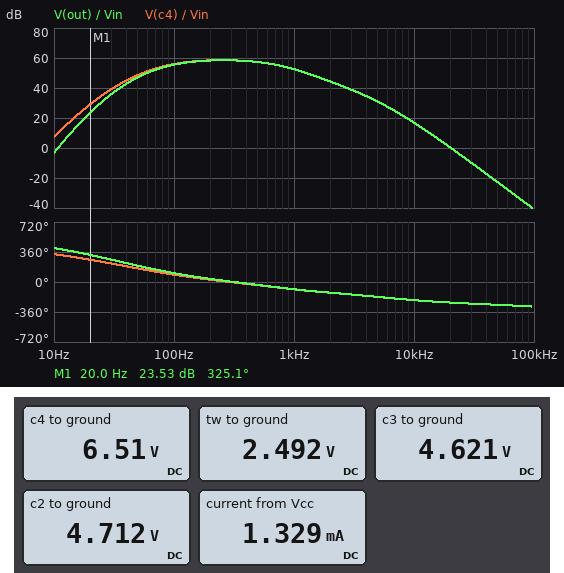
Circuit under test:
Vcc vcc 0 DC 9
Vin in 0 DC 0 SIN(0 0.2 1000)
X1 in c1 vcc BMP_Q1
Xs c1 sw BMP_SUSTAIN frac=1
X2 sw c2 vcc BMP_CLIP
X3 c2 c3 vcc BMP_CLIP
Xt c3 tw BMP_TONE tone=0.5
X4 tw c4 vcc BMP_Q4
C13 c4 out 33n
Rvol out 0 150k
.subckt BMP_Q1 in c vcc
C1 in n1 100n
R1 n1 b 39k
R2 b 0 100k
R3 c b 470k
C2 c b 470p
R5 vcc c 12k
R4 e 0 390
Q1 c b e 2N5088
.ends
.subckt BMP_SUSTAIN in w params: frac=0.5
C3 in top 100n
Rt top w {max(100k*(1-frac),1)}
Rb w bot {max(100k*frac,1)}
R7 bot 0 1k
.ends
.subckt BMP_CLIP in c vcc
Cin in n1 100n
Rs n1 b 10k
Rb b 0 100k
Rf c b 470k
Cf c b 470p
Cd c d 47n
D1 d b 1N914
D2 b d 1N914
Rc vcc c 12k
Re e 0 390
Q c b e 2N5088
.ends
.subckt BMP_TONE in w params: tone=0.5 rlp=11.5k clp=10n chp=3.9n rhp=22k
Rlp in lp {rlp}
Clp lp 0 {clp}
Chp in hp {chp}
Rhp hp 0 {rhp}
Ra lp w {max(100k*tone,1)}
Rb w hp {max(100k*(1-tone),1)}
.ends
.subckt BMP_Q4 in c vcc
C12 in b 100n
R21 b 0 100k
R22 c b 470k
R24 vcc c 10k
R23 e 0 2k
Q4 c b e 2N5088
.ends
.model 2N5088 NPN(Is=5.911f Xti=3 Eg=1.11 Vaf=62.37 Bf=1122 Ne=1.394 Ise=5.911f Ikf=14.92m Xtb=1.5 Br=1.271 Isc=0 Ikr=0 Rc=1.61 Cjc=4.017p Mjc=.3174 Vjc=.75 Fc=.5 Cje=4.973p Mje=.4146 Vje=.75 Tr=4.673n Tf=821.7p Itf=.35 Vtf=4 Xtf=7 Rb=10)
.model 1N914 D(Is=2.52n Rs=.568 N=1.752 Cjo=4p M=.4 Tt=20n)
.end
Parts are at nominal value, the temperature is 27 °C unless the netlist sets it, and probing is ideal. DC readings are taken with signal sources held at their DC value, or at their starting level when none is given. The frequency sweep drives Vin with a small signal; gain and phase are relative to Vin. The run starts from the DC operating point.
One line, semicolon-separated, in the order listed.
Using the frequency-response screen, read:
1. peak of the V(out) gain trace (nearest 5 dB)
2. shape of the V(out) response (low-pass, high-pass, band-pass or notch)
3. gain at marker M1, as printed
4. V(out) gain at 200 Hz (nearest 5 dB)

60 dB; band-pass; 23.53 dB; 60 dB
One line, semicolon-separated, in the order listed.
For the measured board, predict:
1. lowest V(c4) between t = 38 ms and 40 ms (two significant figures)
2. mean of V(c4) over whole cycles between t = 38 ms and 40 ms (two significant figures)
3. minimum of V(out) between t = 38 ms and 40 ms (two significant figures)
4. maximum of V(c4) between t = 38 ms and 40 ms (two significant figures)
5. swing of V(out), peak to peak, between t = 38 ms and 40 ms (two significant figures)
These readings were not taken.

5.8 V; 6.5 V; -660 mV; 7.2 V; 1.3 V
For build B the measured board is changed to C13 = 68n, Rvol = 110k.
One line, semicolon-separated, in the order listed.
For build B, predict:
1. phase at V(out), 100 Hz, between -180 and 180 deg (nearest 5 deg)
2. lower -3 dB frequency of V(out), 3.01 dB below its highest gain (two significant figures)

100 deg; 97 Hz
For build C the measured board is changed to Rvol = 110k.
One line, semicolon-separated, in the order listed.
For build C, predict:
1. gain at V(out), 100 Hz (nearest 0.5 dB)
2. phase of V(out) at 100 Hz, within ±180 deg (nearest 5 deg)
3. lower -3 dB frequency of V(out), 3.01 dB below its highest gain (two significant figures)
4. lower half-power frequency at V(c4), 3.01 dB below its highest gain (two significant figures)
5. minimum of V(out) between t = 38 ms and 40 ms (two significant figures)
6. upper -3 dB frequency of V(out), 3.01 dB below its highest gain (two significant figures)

55.0 dB; 110 deg; 100 Hz; 93 Hz; -640 mV; 710 Hz
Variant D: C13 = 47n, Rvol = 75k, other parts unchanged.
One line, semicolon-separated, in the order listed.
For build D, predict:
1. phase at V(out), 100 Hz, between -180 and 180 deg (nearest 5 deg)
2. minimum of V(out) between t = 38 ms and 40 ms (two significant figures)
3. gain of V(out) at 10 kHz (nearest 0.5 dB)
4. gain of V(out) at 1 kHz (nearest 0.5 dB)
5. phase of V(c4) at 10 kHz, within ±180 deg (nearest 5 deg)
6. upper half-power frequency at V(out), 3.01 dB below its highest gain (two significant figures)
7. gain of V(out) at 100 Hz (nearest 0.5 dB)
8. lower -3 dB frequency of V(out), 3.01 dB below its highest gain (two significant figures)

110 deg; -620 mV; 16.5 dB; 52.0 dB; 140 deg; 710 Hz; 55.0 dB; 100 Hz
